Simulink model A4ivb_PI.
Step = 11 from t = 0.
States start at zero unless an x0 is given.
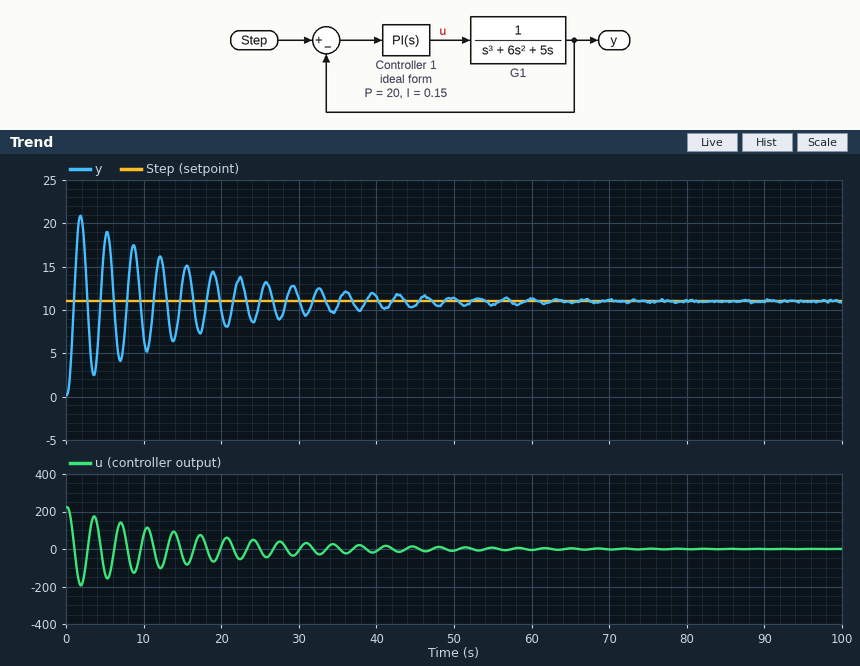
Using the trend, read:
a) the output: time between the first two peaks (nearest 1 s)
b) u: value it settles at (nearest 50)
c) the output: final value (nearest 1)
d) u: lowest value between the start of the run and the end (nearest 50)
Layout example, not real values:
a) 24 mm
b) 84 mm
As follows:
a) 3 s
b) 0
c) 11
d) -200
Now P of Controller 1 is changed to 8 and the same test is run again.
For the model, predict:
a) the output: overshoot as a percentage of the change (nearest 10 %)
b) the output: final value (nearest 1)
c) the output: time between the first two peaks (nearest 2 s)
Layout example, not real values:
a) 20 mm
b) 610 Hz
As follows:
a) 60 %
b) 11
c) 6 s
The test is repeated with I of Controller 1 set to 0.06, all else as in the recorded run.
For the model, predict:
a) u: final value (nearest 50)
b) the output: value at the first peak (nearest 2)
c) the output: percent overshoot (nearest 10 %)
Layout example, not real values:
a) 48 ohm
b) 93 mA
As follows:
a) 0
b) 20
c) 80 %
